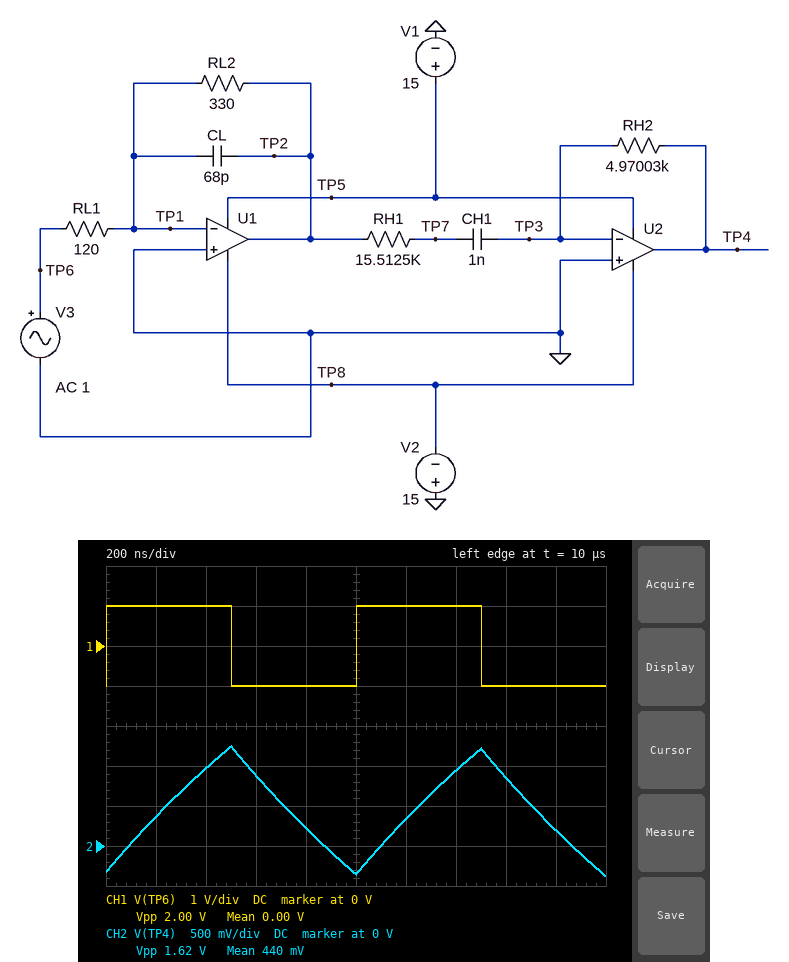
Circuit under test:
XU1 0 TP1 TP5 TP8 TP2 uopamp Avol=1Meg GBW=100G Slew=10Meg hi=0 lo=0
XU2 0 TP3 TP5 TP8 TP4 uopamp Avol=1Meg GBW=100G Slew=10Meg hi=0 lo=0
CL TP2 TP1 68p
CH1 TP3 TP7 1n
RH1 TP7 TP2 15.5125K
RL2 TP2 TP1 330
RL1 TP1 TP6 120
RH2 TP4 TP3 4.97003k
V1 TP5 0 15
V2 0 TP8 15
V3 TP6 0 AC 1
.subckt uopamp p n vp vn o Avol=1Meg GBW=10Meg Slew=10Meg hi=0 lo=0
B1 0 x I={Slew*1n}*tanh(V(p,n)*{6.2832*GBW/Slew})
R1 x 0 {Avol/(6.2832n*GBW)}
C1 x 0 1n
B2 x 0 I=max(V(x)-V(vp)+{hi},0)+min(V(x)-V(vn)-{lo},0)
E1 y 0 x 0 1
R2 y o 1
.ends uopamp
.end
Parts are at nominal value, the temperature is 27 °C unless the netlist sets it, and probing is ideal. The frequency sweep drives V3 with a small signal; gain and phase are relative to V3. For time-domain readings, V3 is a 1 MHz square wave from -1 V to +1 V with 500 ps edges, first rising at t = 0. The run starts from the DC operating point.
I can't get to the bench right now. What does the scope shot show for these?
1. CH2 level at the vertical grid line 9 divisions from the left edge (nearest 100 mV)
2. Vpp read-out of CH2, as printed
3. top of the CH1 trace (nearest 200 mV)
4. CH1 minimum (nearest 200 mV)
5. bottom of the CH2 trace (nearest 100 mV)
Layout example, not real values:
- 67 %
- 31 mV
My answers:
- 200 mV
- 1.62 V
- 1.0 V
- -1.0 V
- -400 mV
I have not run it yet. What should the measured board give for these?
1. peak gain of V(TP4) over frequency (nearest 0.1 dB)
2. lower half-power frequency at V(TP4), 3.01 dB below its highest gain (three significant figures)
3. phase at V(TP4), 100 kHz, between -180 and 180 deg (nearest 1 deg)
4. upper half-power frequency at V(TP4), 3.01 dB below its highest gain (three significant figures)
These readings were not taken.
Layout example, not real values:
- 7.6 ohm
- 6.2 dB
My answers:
- -1.1 dB
- 10.2 kHz
- 5 deg
- 7.11 MHz
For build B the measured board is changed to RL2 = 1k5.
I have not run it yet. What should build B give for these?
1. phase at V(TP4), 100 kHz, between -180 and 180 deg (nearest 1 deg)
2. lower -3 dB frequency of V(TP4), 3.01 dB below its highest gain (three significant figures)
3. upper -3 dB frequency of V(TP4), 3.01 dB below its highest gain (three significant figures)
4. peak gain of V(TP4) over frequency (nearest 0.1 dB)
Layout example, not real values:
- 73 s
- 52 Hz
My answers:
- 2 deg
- 10.1 kHz
- 1.58 MHz
- 12.0 dB
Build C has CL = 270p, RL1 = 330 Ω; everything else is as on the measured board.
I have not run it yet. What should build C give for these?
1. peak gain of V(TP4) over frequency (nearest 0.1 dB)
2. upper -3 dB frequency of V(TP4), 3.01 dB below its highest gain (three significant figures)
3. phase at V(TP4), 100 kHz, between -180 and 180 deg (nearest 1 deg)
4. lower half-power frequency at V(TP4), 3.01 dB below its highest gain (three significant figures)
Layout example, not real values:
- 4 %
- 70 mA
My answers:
- -9.9 dB
- 1.81 MHz
- 3 deg
- 10.1 kHz
